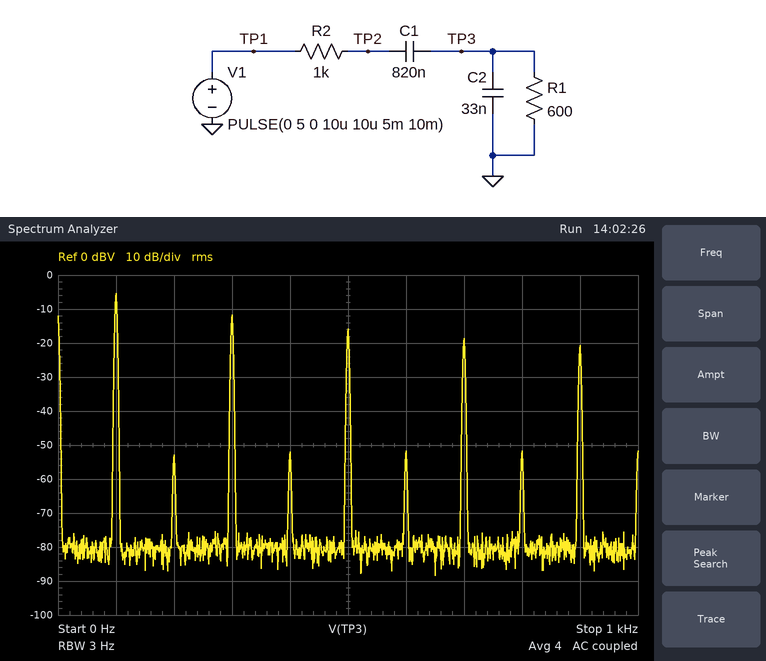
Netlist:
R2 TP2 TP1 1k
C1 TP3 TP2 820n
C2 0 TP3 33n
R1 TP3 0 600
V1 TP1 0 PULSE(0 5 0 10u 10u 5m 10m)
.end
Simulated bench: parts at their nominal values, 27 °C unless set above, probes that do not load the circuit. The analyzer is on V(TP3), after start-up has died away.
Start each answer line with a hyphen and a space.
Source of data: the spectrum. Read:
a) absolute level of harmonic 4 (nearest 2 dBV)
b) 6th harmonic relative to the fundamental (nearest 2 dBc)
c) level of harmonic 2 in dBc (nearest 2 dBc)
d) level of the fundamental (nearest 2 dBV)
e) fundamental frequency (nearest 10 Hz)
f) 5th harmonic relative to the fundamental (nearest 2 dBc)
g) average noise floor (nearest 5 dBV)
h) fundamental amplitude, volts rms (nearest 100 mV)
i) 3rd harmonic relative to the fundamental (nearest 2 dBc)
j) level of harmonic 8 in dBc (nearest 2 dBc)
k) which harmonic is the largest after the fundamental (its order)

- -52 dBV
- -46 dBc
- -48 dBc
- -6 dBV
- 100 Hz
- -10 dBc
- -80 dBV
- 500 mV
- -6 dBc
- -46 dBc
- 3
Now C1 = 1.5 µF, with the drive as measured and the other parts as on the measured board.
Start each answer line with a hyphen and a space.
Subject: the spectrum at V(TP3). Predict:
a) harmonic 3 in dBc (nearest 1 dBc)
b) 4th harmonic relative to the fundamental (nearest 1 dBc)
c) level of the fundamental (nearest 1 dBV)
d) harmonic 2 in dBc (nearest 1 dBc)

- -8 dBc
- -49 dBc
- -3 dBV
- -49 dBc
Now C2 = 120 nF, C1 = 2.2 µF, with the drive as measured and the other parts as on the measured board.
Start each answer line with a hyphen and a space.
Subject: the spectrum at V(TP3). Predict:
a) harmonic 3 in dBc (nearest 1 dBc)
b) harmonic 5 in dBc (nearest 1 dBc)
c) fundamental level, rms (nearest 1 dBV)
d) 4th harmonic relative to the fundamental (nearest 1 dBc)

- -9 dBc
- -13 dBc
- -2 dBV
- -49 dBc
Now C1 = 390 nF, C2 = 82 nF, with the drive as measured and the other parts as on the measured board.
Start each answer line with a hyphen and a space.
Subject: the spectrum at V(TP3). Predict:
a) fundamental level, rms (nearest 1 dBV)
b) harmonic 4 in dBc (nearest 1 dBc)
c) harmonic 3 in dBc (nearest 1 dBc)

- -10 dBV
- -43 dBc
- -3 dBc
